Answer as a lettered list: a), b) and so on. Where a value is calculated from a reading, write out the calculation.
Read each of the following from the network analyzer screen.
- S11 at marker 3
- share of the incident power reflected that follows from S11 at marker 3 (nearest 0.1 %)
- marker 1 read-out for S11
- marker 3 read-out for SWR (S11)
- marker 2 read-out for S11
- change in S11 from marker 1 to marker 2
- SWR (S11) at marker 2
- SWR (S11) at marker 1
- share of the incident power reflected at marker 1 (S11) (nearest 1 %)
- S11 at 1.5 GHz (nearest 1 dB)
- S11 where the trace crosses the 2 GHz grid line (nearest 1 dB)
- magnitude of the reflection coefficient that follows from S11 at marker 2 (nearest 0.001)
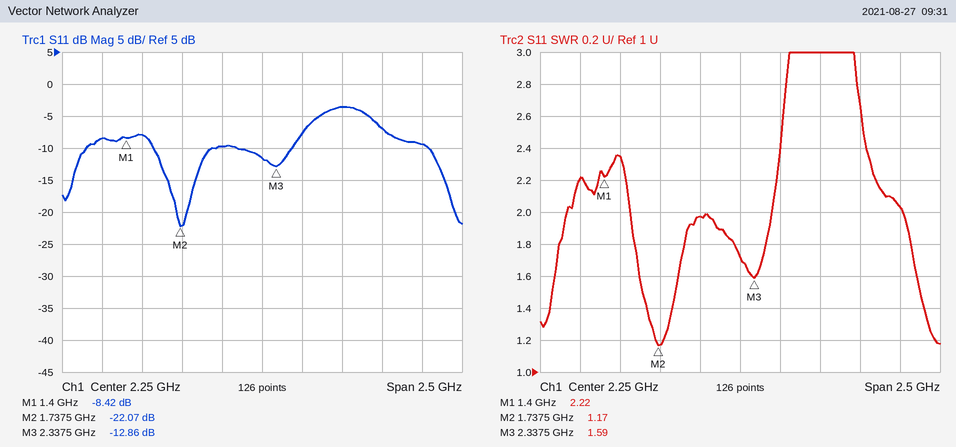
a) -12.86 dB
b) 10^(-12.86/10) ≈ 5.2 %
c) -8.42 dB
d) 1.59
e) -22.07 dB
f) -22.07 − (-8.42) = -13.65 dB
g) 1.17
h) 2.22
i) 10^(-8.42/10) ≈ 14 %
j) -8 dB
k) -10 dB
l) 10^(-22.07/20) ≈ 0.079
